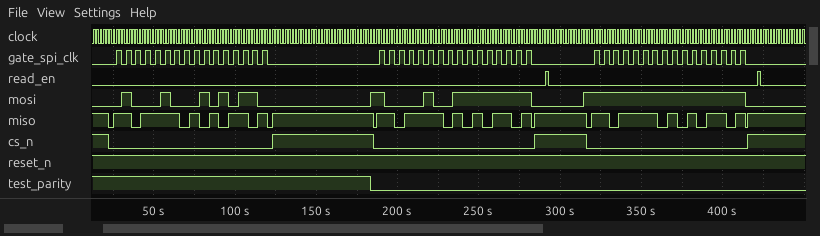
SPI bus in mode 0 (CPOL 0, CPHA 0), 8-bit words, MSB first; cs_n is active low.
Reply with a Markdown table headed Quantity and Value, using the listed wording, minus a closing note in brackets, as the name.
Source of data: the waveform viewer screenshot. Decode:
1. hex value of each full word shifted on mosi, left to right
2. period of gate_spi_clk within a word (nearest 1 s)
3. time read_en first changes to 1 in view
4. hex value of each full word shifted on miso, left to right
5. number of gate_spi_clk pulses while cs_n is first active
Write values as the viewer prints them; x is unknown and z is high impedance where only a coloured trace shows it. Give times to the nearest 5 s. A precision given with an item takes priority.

| Quantity | Value |
|---|---|
| hex value of each full word shifted on mosi, left to right | 44, 56, 84, FF, FF, FF |
| period of gate_spi_clk within a word | 6 s |
| time read_en first changes to 1 in view | 290 s |
| hex value of each full word shifted on miso, left to right | DE, AD, DE, AD, DE, AD |
| number of gate_spi_clk pulses while cs_n is first active | 16 |
